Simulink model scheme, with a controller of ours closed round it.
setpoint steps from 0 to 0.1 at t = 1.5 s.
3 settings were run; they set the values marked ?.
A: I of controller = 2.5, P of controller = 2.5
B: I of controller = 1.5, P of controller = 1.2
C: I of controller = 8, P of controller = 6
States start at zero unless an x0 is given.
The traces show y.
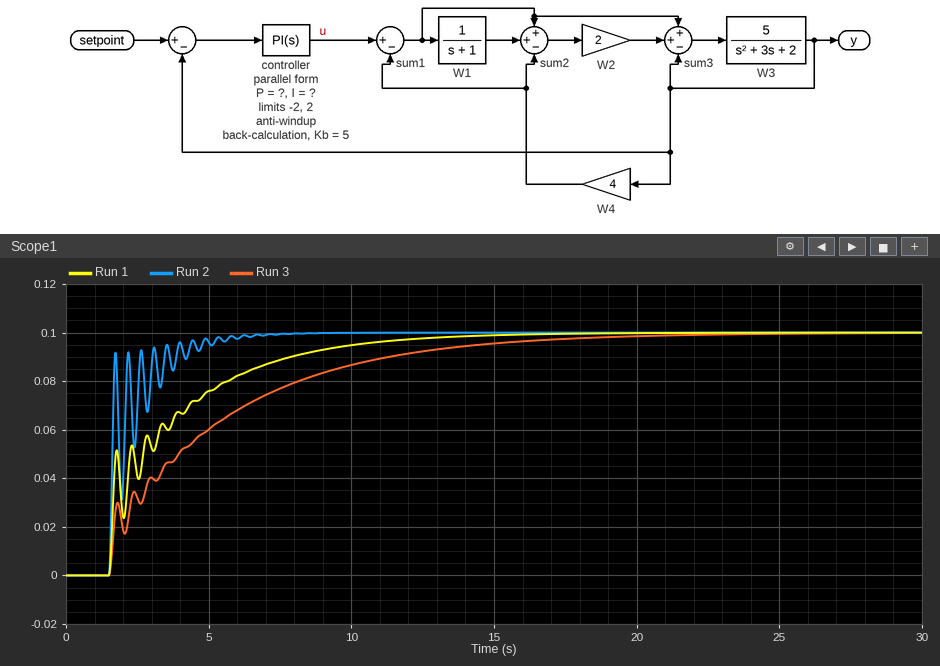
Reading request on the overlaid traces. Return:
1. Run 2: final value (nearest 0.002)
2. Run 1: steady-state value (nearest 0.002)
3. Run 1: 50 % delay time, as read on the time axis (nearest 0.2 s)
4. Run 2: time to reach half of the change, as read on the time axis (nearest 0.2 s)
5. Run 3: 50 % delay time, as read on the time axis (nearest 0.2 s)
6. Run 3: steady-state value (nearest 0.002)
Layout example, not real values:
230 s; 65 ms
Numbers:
0.100; 0.100; 1.8 s; 1.6 s; 4.0 s; 0.100
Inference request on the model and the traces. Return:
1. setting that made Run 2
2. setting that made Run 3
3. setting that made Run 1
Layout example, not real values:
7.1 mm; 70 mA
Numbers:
C; B; A
